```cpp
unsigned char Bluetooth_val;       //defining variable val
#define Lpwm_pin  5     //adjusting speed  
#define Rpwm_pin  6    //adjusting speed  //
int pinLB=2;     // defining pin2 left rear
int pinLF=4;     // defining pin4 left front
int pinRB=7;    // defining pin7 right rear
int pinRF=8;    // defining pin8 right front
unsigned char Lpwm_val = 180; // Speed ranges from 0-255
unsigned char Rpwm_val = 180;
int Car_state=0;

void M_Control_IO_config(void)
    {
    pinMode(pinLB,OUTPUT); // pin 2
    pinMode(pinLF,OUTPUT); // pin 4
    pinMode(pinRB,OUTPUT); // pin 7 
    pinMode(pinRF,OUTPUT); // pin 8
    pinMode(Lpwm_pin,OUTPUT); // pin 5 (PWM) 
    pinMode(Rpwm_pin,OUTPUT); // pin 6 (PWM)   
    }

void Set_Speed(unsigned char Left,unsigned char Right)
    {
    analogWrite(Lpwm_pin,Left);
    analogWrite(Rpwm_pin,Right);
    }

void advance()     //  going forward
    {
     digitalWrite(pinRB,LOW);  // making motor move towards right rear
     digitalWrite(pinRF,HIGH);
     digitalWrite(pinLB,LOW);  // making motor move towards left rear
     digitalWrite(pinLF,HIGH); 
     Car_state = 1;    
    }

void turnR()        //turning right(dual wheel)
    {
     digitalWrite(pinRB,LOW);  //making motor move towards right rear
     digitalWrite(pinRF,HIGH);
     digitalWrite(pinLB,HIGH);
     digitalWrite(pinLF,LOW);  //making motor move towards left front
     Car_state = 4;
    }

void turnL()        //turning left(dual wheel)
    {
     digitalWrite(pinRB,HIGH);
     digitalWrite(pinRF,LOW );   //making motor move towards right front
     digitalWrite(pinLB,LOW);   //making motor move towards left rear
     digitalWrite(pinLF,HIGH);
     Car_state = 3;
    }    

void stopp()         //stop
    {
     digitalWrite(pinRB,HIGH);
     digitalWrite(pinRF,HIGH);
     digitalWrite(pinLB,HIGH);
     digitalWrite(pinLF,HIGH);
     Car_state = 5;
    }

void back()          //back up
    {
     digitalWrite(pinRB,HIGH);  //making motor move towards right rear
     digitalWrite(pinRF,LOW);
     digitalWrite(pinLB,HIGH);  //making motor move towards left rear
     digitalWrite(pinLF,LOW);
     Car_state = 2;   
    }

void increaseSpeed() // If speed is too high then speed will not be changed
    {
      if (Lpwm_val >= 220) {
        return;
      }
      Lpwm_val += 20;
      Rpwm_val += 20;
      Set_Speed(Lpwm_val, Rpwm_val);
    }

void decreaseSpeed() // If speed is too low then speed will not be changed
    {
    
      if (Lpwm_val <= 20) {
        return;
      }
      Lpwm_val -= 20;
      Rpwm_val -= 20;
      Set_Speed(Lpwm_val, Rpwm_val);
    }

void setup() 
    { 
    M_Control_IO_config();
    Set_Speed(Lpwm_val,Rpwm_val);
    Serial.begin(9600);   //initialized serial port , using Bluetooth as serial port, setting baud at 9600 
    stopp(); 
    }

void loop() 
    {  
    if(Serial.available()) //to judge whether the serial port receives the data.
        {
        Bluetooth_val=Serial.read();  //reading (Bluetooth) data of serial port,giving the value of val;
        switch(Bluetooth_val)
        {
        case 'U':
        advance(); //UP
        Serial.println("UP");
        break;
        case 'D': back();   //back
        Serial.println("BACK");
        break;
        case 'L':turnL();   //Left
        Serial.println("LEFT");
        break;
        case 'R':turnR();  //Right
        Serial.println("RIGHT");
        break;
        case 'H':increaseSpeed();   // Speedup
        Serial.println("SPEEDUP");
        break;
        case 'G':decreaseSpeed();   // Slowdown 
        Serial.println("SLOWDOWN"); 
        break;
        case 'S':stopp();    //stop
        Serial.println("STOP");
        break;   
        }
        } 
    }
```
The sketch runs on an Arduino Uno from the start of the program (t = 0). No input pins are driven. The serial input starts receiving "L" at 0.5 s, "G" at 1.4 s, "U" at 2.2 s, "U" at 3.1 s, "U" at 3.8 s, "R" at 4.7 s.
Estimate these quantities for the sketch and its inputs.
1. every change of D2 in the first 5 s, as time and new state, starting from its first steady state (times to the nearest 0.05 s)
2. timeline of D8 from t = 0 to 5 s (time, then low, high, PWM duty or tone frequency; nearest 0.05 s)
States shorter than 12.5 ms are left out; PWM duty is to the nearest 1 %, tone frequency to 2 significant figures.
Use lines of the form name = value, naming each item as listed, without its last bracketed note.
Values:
every change of D2 in the first 5 s, as time and new state, starting from its first steady state = 0 s high; 0.5 s low; 4.7 s high
timeline of D8 from t = 0 to 5 s = 0 s high; 0.5 s low; 2.2 s high
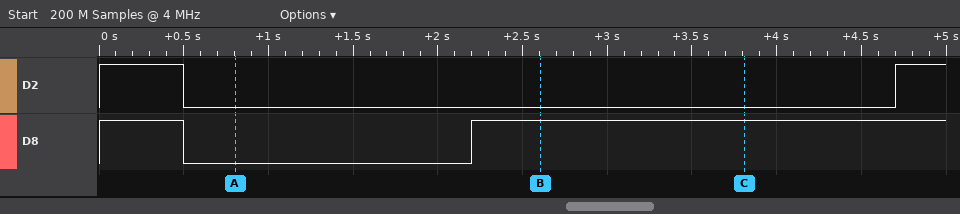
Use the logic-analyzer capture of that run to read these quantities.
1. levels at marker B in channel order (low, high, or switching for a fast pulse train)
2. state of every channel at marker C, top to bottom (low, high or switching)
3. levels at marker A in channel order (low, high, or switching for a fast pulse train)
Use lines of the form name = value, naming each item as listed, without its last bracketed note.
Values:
levels at marker B in channel order = D2 low, D8 high
state of every channel at marker C, top to bottom = D2 low, D8 high
levels at marker A in channel order = D2 low, D8 low
